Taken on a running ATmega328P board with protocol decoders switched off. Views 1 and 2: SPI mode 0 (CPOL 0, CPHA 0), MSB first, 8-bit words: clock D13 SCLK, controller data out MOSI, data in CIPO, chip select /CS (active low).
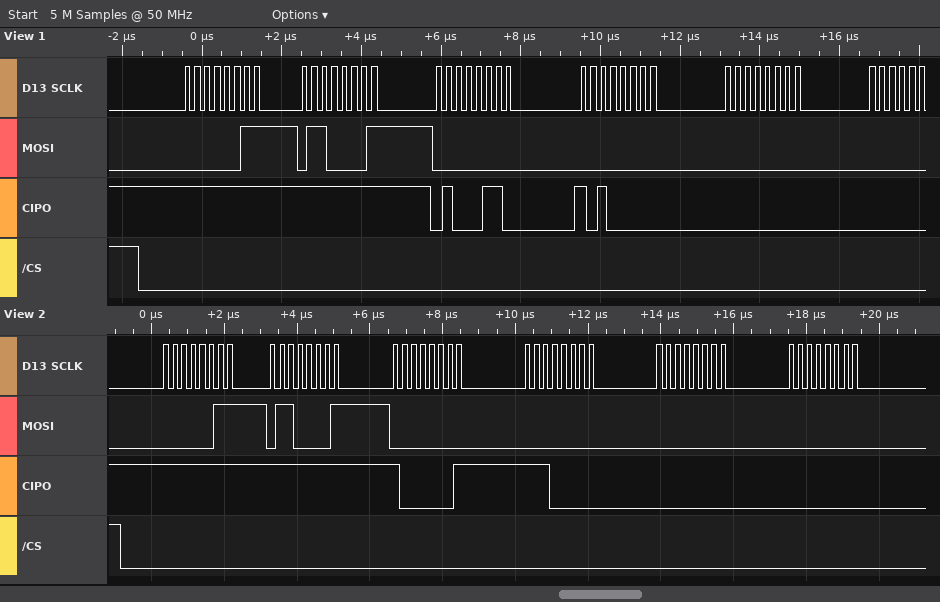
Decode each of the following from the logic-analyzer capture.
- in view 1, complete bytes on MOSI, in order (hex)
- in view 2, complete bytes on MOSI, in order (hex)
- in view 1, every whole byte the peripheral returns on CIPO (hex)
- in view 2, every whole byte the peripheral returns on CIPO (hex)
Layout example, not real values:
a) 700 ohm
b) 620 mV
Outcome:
a) 03 61 00 00 00
b) 03 61 00 00 00 00
c) FF FF 46 A0 00
d) FF FF 81 E0 00 00
